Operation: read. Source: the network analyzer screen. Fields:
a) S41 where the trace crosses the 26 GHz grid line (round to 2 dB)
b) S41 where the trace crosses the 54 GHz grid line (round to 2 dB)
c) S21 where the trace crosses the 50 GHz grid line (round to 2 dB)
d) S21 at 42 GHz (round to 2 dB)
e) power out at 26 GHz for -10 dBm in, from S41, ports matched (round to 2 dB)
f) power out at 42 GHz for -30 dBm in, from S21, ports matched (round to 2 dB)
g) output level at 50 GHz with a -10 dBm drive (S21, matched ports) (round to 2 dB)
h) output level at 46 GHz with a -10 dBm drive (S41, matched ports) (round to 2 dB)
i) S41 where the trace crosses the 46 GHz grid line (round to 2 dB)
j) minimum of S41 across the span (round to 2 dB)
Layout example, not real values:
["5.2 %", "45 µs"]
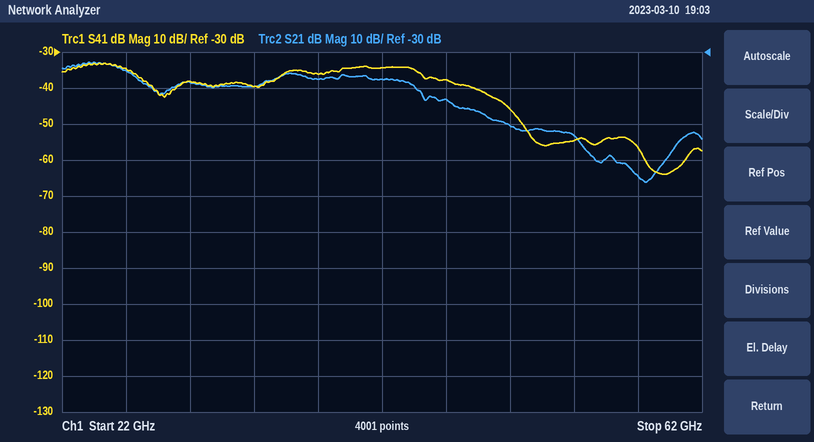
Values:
["-34 dB", "-54 dB", "-50 dB", "-38 dB", "-44 dBm", "-68 dBm", "-60 dBm", "-48 dBm", "-38 dB", "-64 dB"]
